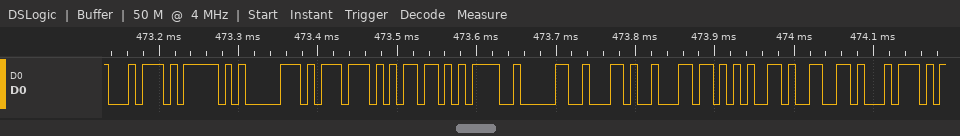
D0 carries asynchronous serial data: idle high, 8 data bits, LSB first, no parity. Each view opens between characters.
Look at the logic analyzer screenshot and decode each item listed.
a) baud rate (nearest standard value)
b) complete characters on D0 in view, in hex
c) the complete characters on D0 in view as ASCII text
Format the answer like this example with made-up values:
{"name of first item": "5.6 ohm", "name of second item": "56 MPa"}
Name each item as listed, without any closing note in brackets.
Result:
{"baud rate": "115200 baud", "complete characters on D0 in view, in hex": "74, 5F, 70, 77, 6D, 3D, 30, 2C, 6C, 65, 66, 74", "the complete characters on D0 in view as ASCII text": "\"t_pwm=0,left\""}
